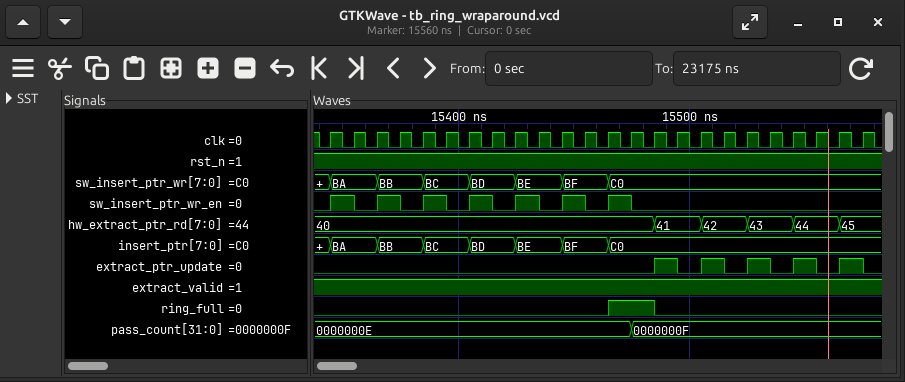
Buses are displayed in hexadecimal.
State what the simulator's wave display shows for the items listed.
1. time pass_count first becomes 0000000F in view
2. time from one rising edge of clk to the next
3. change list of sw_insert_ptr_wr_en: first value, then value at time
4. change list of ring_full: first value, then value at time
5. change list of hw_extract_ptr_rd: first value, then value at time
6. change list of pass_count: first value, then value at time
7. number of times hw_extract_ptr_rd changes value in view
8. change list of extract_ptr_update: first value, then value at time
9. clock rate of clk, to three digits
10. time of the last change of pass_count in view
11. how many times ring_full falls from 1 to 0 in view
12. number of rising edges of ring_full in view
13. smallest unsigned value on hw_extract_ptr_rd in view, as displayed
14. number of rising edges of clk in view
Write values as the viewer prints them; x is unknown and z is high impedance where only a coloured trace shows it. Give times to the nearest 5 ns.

15475 ns
10 ns
0, 1 at 15345 ns, 0 at 15355 ns, 1 at 15365 ns, 0 at 15375 ns, 1 at 15385 ns, 0 at 15395 ns, 1 at 15405 ns, 0 at 15415 ns, 1 at 15425 ns, 0 at 15435 ns, 1 at 15445 ns, 0 at 15455 ns, 1 at 15465 ns, 0 at 15475 ns
0, 1 at 15465 ns, 0 at 15485 ns
40, 41 at 15485 ns, 42 at 15505 ns, 43 at 15525 ns, 44 at 15545 ns, 45 at 15565 ns
0000000E, 0000000F at 15475 ns
5
0, 1 at 15485 ns, 0 at 15495 ns, 1 at 15505 ns, 0 at 15515 ns, 1 at 15525 ns, 0 at 15535 ns, 1 at 15545 ns, 0 at 15555 ns, 1 at 15565 ns, 0 at 15575 ns
100 MHz
15475 ns
1
1
40
24
